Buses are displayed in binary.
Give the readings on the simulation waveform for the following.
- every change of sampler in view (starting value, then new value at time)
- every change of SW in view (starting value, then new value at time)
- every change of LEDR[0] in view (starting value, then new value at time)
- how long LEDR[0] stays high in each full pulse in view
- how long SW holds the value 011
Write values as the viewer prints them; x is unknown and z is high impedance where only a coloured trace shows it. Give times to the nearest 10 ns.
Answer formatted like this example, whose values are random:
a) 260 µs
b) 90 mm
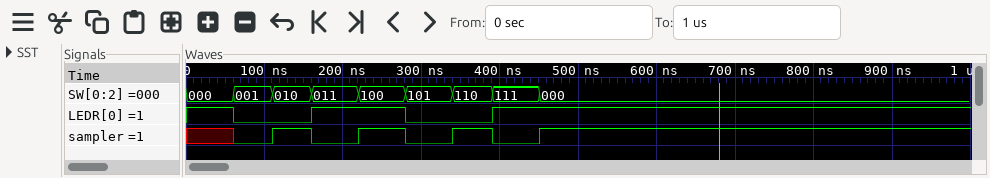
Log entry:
a) x, 0 at 60 ns, 1 at 110 ns, 0 at 160 ns, 1 at 220 ns, 0 at 280 ns, 1 at 340 ns, 0 at 390 ns, 1 at 450 ns
b) 000, 001 at 60 ns, 010 at 110 ns, 011 at 160 ns, 100 at 220 ns, 101 at 280 ns, 110 at 340 ns, 111 at 390 ns, 000 at 450 ns
c) 1, 0 at 60 ns, 1 at 160 ns, 0 at 280 ns, 1 at 390 ns
d) 120 ns
e) 60 ns
